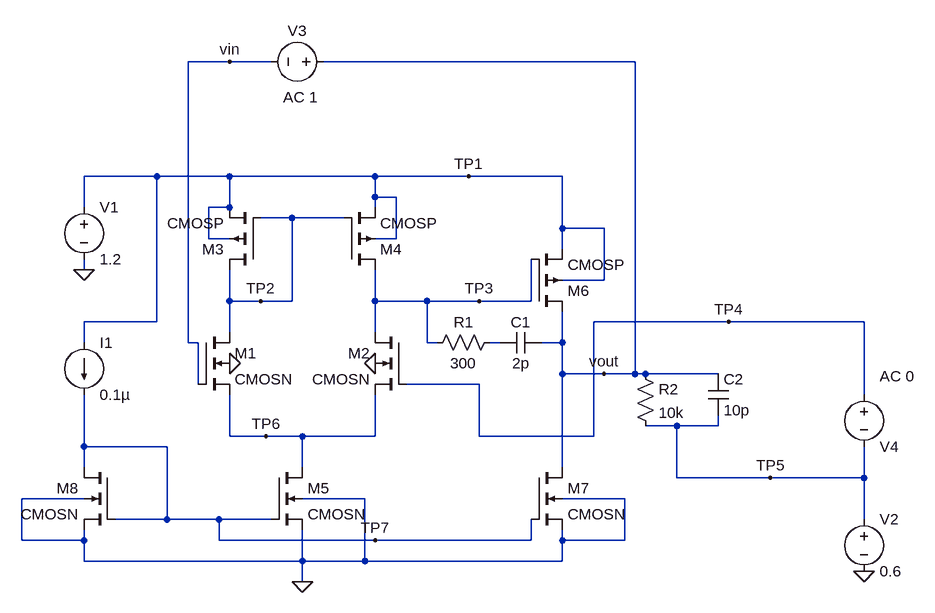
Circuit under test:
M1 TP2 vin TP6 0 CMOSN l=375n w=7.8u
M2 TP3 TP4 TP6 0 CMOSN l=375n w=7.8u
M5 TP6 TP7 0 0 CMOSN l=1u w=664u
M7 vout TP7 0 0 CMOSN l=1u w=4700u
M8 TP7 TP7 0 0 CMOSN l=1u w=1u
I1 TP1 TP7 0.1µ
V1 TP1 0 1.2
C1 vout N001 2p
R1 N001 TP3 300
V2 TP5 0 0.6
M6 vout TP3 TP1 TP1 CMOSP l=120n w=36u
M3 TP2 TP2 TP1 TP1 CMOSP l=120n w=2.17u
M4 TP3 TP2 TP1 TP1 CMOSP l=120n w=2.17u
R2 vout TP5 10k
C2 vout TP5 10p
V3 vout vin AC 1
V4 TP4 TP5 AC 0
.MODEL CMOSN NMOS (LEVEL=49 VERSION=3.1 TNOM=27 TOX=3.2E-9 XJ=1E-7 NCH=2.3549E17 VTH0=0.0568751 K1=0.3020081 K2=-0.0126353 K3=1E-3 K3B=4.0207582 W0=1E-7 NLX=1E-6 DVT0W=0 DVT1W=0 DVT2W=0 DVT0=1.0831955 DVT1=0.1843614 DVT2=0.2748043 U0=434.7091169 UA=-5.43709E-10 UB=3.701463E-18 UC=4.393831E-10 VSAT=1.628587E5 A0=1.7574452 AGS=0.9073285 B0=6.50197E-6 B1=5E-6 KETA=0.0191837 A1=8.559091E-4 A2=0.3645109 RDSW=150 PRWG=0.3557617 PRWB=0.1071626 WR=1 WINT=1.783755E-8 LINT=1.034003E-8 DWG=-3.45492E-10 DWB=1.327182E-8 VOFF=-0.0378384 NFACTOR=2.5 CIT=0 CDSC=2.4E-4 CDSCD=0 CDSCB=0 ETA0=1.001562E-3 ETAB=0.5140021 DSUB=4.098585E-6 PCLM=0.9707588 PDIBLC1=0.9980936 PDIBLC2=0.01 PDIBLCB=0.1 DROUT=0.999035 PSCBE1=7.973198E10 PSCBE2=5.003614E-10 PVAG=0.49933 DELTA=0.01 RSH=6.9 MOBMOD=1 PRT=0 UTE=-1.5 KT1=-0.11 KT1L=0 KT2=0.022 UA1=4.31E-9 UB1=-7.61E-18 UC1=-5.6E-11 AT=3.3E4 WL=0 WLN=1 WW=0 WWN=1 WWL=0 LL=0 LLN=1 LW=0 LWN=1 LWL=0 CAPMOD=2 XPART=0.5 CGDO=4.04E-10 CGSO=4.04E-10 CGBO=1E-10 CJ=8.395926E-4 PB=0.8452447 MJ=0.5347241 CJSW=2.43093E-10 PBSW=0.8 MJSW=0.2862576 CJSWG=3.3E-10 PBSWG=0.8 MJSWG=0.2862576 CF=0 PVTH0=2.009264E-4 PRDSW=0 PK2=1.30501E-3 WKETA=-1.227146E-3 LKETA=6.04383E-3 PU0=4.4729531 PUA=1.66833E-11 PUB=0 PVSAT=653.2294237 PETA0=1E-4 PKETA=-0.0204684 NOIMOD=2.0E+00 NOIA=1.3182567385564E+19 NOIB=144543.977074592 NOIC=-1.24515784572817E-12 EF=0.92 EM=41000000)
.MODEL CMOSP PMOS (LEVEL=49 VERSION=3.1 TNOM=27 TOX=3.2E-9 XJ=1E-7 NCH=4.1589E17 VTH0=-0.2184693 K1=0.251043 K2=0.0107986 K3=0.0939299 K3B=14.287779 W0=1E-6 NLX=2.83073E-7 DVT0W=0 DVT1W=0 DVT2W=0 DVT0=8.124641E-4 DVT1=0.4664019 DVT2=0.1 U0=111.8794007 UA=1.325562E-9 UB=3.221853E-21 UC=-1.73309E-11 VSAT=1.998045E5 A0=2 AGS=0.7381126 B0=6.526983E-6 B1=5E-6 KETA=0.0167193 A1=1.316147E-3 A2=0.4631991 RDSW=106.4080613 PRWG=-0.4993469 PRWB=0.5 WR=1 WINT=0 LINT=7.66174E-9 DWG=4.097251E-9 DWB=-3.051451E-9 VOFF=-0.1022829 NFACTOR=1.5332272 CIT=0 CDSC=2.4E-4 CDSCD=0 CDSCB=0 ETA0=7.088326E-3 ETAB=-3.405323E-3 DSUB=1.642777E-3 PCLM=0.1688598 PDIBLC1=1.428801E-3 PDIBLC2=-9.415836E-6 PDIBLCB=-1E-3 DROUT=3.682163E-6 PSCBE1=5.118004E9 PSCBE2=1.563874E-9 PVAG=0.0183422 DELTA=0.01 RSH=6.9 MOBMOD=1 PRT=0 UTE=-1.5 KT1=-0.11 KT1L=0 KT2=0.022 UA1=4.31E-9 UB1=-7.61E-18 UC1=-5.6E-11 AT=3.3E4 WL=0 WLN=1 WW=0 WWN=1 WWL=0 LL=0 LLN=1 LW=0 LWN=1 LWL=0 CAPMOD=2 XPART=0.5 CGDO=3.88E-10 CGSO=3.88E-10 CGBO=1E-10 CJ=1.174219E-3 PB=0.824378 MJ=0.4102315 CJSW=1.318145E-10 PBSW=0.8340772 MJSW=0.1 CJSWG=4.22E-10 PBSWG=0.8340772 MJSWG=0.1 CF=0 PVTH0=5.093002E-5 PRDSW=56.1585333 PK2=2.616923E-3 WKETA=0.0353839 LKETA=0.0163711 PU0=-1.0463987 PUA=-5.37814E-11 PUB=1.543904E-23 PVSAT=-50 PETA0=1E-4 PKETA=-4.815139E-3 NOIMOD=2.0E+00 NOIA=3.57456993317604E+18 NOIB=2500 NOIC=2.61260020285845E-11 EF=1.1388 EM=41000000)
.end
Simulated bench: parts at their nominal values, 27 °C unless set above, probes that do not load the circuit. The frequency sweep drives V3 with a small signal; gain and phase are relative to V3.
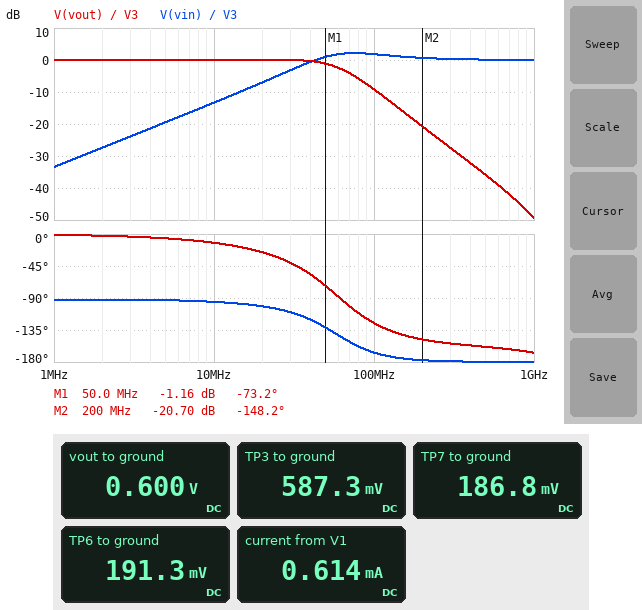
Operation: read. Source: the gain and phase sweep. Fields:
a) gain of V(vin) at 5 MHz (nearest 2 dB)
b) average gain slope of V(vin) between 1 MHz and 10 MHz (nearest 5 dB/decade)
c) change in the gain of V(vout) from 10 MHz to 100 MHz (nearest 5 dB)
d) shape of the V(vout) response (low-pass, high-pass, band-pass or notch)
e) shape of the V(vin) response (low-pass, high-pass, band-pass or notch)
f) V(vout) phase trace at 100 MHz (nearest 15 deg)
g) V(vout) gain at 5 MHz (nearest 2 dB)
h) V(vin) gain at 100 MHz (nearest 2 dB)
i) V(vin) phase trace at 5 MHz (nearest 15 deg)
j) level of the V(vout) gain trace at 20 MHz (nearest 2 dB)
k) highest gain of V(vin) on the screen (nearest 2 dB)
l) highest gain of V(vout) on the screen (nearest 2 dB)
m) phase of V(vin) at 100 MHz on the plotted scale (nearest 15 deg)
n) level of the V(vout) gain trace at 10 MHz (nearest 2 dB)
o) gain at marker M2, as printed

-20 dB
20 dB/decade
-10 dB
low-pass
high-pass
-120 deg
0 dB
2 dB
-90 deg
0 dB
2 dB
0 dB
-165 deg
0 dB
-20.70 dB
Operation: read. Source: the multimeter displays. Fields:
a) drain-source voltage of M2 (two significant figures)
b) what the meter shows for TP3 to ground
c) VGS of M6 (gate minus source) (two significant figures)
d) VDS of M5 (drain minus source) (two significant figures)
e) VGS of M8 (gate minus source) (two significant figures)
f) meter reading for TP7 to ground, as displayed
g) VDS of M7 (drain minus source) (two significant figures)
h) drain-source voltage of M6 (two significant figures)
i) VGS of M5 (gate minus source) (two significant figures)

400 mV
587.3 mV
-610 mV
190 mV
190 mV
186.8 mV
600 mV
-600 mV
190 mV
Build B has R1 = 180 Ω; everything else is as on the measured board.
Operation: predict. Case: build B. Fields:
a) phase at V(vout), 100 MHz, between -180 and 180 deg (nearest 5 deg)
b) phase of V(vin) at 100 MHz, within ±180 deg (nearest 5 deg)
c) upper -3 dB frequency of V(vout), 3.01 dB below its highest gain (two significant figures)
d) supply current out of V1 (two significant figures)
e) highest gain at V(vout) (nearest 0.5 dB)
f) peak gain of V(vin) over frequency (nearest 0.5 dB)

-135 deg
-170 deg
65 MHz
610 µA
0.5 dB
2.5 dB
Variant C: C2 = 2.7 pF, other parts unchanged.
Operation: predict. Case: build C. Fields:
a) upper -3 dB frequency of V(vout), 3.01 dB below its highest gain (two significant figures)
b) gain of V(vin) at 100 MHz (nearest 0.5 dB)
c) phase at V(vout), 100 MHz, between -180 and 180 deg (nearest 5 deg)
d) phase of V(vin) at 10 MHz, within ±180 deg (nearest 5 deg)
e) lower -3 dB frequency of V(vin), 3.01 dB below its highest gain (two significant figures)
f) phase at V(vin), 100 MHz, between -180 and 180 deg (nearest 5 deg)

59 MHz
1.0 dB
-90 deg
-100 deg
46 MHz
-155 deg
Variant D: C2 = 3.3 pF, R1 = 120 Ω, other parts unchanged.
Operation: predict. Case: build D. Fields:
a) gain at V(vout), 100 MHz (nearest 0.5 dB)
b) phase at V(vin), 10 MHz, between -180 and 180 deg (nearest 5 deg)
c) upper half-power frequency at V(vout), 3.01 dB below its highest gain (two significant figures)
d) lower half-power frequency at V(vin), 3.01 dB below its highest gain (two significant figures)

-6.0 dB
-100 deg
69 MHz
47 MHz
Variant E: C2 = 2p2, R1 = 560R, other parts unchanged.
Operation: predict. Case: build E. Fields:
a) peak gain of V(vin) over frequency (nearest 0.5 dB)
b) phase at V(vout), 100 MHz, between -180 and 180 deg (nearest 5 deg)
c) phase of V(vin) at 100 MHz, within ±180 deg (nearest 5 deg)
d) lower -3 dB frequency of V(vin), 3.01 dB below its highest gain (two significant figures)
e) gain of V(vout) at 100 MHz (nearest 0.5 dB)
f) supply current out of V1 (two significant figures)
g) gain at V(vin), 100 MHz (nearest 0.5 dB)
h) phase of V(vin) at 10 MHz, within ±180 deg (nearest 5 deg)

0 dB
-70 deg
-155 deg
47 MHz
-7.0 dB
610 µA
-0.5 dB
-100 deg
